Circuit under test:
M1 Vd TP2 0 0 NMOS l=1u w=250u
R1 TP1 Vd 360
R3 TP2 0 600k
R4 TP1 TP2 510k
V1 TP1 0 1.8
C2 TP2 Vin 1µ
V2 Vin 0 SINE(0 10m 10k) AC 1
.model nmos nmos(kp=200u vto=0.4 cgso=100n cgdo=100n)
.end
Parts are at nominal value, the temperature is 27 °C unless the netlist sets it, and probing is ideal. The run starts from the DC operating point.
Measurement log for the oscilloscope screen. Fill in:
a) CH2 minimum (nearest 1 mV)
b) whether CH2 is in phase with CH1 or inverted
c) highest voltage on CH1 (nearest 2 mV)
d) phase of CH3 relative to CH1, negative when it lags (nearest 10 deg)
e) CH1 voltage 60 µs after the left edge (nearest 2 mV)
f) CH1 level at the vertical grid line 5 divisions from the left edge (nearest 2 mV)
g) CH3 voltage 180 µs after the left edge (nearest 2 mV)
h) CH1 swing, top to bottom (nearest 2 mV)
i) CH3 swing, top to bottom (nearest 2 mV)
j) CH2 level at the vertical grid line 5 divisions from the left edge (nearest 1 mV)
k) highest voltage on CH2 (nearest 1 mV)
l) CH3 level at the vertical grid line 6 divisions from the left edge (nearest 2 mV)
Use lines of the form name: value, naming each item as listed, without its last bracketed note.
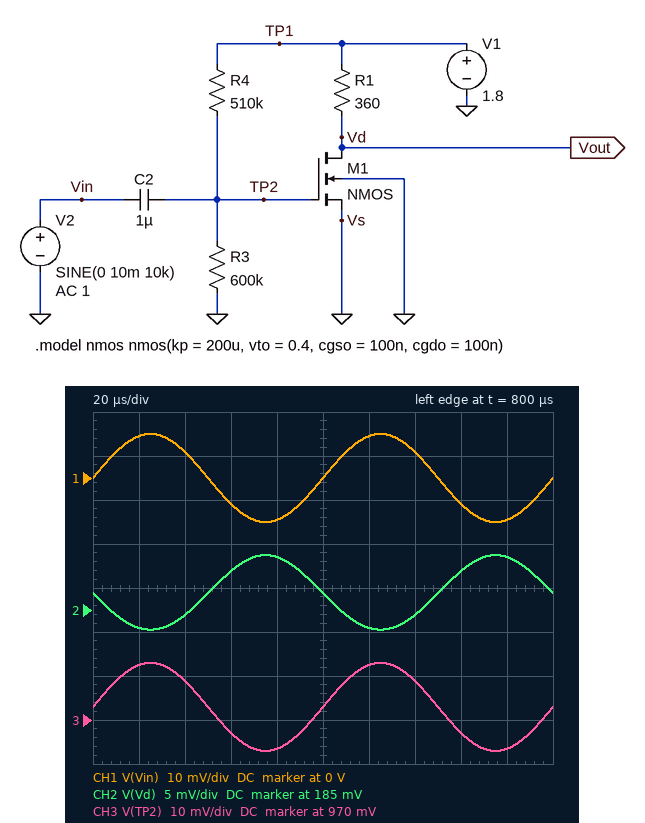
CH2 minimum: 183 mV
whether CH2 is in phase with CH1 or inverted: inverted
highest voltage on CH1: 10 mV
phase of CH3 relative to CH1, negative when it lags: 0 deg
CH1 voltage 60 µs after the left edge: -6 mV
CH1 level at the vertical grid line 5 divisions from the left edge: 0 V
CH3 voltage 180 µs after the left edge: 964 mV
CH1 swing, top to bottom: 20 mV
CH3 swing, top to bottom: 20 mV
CH2 level at the vertical grid line 5 divisions from the left edge: 187 mV
highest voltage on CH2: 191 mV
CH3 level at the vertical grid line 6 divisions from the left edge: 982 mV
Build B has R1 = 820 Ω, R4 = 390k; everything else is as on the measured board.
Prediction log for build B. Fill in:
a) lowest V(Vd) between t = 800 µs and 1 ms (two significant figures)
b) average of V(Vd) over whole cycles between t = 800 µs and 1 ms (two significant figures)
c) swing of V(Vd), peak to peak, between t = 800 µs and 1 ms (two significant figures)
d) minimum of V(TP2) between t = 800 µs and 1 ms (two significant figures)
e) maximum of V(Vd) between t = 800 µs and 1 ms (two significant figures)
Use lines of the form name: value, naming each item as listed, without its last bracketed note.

lowest V(Vd) between t = 800 µs and 1 ms: 63 mV
average of V(Vd) over whole cycles between t = 800 µs and 1 ms: 64 mV
swing of V(Vd), peak to peak, between t = 800 µs and 1 ms: 2.0 mV
minimum of V(TP2) between t = 800 µs and 1 ms: 1.1 V
maximum of V(Vd) between t = 800 µs and 1 ms: 65 mV
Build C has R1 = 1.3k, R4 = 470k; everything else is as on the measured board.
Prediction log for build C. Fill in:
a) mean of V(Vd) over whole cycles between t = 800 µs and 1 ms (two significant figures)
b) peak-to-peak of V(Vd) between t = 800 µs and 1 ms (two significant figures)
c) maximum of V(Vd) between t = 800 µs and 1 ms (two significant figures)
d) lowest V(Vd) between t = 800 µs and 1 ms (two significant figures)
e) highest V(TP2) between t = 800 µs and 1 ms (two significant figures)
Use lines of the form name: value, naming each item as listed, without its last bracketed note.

mean of V(Vd) over whole cycles between t = 800 µs and 1 ms: 46 mV
peak-to-peak of V(Vd) between t = 800 µs and 1 ms: 1.6 mV
maximum of V(Vd) between t = 800 µs and 1 ms: 47 mV
lowest V(Vd) between t = 800 µs and 1 ms: 45 mV
highest V(TP2) between t = 800 µs and 1 ms: 1.0 V
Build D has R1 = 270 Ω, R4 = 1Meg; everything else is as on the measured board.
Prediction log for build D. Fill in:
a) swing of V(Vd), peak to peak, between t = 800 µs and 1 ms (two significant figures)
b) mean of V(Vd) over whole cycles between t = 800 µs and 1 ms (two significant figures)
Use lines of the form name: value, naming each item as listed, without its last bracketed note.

swing of V(Vd), peak to peak, between t = 800 µs and 1 ms: 74 mV
mean of V(Vd) over whole cycles between t = 800 µs and 1 ms: 1.3 V
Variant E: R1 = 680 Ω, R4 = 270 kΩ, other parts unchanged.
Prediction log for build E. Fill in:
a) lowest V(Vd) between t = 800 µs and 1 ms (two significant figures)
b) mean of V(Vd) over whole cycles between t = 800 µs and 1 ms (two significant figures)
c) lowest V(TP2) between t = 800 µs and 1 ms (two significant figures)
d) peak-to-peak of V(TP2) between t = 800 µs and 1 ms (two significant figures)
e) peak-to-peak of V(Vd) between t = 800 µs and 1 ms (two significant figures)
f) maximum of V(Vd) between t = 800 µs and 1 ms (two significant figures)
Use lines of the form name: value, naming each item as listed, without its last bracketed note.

lowest V(Vd) between t = 800 µs and 1 ms: 62 mV
mean of V(Vd) over whole cycles between t = 800 µs and 1 ms: 63 mV
lowest V(TP2) between t = 800 µs and 1 ms: 1.2 V
peak-to-peak of V(TP2) between t = 800 µs and 1 ms: 20 mV
peak-to-peak of V(Vd) between t = 800 µs and 1 ms: 1.6 mV
maximum of V(Vd) between t = 800 µs and 1 ms: 64 mV
